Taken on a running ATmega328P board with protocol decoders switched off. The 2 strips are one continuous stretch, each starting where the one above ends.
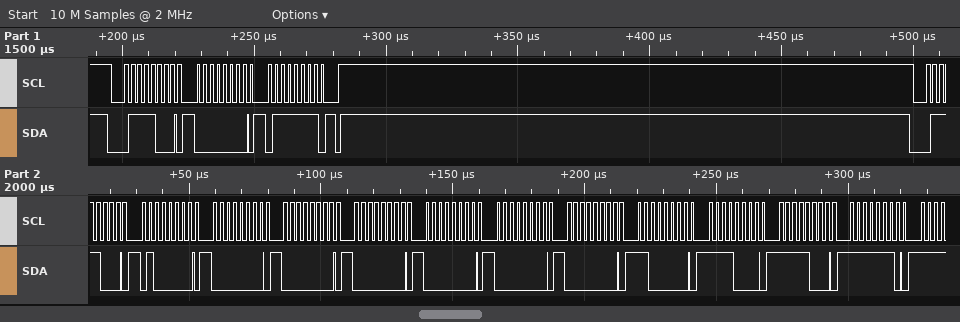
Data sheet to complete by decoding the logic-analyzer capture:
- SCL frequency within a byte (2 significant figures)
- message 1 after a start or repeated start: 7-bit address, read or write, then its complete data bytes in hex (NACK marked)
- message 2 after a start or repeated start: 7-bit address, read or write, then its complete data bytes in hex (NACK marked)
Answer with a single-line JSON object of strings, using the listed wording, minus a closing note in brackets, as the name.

{"SCL frequency within a byte": "400 kHz", "message 1 after a start or repeated start: 7-bit address, read or write, then its complete data bytes in hex": "0x3C write: 00 7F", "message 2 after a start or repeated start: 7-bit address, read or write, then its complete data bytes in hex": "0x3C write: 40 00 00 00 00 00 00 C0 F0 F8 FE"}
